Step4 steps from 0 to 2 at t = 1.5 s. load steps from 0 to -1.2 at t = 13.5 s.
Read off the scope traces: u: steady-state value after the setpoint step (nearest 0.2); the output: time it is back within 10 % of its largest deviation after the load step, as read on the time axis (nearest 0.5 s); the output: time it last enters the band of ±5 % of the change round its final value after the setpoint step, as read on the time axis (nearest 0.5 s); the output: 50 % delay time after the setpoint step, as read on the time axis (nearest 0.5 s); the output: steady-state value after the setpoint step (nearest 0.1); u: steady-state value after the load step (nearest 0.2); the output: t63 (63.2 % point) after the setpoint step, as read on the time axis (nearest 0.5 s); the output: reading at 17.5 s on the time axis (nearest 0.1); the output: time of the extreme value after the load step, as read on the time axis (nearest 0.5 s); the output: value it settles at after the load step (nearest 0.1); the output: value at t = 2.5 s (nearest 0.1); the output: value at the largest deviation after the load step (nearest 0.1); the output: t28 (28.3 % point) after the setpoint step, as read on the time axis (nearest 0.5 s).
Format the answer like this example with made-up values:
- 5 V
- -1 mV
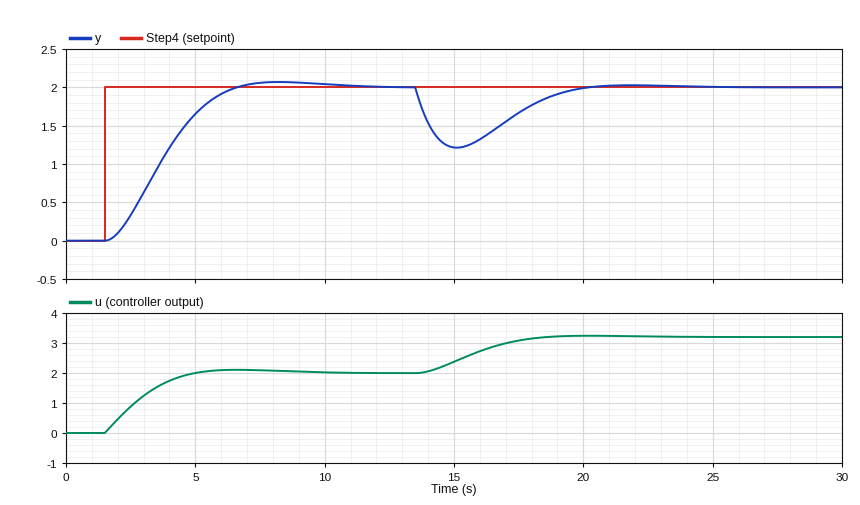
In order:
- 2.0
- 19.0 s
- 6.0 s
- 3.5 s
- 2.0
- 3.2
- 4.0 s
- 1.7
- 15.0 s
- 2.0
- 0.3
- 1.2
- 3.0 s
